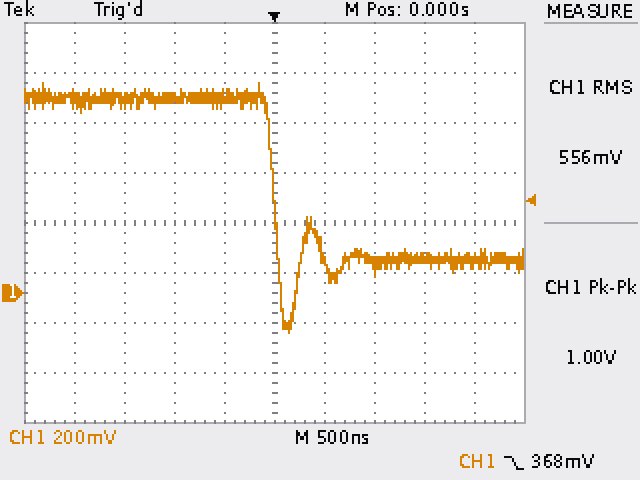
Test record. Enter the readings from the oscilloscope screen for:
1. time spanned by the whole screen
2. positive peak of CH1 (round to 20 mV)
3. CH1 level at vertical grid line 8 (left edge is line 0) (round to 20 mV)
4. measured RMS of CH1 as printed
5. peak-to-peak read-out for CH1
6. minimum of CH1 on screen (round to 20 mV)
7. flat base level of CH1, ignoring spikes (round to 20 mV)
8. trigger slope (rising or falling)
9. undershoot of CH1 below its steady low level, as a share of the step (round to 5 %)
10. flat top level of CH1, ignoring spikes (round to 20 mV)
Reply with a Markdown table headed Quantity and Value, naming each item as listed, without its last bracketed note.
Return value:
| Quantity | Value |
|---|---|
| time spanned by the whole screen | 5 µs |
| positive peak of CH1 | 840 mV |
| CH1 level at vertical grid line 8 (left edge is line 0) | 140 mV |
| measured RMS of CH1 as printed | 556 mV |
| peak-to-peak read-out for CH1 | 1.00 V |
| minimum of CH1 on screen | -160 mV |
| flat base level of CH1, ignoring spikes | 140 mV |
| trigger slope | falling |
| undershoot of CH1 below its steady low level, as a share of the step | 45 % |
| flat top level of CH1, ignoring spikes | 780 mV |
